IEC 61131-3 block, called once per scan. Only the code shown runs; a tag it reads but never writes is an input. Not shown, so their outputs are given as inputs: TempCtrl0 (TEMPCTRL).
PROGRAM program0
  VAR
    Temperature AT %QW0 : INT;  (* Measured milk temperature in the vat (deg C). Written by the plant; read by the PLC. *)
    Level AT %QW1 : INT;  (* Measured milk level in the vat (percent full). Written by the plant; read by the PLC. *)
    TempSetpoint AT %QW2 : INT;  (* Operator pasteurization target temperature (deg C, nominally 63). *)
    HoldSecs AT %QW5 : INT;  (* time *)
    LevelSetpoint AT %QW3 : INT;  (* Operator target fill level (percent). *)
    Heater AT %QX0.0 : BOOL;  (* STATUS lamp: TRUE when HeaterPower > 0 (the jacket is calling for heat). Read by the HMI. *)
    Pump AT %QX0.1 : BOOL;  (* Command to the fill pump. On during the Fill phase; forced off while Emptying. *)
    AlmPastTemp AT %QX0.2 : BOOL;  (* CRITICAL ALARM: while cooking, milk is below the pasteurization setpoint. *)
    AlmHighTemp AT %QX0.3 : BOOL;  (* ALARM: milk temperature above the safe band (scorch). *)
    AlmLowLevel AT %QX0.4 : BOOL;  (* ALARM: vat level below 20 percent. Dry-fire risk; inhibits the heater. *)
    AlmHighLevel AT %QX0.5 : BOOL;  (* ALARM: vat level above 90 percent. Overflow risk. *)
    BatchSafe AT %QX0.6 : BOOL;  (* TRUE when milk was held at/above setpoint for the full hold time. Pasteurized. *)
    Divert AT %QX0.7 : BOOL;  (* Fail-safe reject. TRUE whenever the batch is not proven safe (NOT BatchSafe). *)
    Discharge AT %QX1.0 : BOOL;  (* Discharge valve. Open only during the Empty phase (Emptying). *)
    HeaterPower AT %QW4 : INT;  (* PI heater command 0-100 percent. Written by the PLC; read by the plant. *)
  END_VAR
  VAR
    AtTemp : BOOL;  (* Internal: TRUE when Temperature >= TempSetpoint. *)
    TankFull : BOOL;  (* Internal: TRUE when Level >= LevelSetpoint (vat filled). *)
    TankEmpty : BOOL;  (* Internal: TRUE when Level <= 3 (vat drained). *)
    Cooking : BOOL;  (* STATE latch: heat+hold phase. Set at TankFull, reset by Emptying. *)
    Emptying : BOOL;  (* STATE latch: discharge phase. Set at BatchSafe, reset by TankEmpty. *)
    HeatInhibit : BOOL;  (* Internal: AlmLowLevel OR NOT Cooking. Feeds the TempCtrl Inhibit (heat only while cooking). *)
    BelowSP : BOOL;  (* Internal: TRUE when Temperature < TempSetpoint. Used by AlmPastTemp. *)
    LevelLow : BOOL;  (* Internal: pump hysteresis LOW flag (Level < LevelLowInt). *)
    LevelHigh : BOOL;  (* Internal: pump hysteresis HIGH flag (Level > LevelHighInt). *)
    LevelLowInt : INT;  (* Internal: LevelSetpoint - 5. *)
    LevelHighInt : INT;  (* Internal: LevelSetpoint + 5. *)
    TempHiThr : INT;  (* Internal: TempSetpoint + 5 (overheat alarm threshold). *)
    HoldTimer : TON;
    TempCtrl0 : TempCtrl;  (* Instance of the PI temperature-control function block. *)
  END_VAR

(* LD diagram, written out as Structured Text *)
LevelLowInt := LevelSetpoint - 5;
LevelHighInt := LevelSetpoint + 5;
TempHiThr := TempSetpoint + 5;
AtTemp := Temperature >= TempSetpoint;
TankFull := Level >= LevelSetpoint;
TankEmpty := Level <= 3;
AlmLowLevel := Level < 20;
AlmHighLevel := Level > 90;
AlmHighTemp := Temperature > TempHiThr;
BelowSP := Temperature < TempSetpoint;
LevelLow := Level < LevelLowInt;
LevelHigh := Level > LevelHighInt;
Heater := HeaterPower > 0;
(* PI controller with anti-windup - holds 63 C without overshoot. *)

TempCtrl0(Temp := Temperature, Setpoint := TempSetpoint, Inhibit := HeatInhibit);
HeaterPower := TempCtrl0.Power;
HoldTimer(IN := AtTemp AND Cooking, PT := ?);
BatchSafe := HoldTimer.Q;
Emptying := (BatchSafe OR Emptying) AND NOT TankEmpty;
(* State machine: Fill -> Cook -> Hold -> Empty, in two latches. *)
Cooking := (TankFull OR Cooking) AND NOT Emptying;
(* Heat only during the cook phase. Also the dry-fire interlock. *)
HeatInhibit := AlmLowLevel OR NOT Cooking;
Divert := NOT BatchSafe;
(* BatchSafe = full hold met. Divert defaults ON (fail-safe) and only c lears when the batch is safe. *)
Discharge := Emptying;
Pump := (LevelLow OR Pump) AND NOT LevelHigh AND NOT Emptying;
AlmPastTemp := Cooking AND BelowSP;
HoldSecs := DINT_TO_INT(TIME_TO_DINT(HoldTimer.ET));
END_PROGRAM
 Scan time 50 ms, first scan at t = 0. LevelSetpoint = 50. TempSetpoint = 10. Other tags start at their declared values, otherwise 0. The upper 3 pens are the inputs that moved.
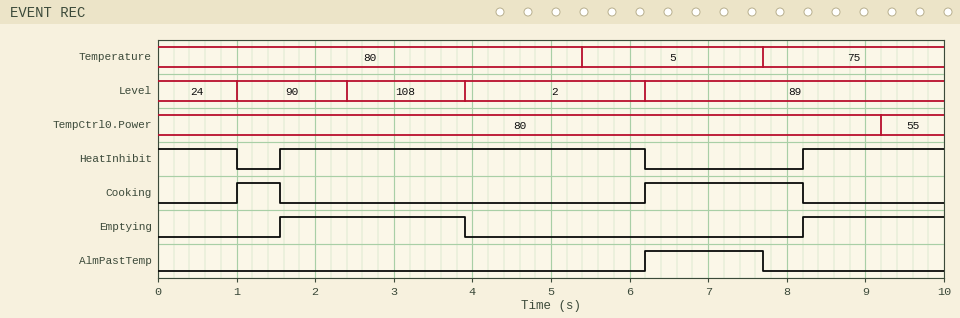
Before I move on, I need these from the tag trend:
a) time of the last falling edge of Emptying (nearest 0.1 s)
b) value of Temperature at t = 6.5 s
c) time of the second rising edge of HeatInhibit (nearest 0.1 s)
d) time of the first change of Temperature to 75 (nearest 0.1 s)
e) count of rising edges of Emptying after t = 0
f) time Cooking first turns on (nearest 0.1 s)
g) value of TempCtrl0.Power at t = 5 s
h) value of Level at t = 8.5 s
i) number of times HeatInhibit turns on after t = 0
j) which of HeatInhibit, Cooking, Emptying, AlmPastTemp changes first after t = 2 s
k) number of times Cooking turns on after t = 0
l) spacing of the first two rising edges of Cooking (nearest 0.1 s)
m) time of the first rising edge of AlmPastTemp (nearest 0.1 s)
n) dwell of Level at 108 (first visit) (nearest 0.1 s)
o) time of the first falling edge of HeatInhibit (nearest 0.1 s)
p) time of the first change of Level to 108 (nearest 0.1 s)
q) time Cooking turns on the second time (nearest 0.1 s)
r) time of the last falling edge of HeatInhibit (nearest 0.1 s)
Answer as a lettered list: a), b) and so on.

a) 3.9 s
b) 5
c) 8.2 s
d) 7.7 s
e) 2
f) 1.0 s
g) 80
h) 89
i) 2
j) Emptying
k) 2
l) 5.2 s
m) 6.2 s
n) 1.5 s
o) 1.0 s
p) 2.4 s
q) 6.2 s
r) 6.2 s
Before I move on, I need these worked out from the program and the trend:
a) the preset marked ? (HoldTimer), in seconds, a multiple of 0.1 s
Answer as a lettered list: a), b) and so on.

a) 0.5 s
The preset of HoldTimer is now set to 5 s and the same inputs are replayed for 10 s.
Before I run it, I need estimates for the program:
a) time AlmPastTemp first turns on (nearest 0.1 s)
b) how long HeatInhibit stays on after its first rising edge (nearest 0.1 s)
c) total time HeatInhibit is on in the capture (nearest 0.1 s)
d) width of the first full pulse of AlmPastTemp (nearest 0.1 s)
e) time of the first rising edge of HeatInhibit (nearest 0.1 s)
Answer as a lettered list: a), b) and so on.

a) 5.4 s
b) 2.3 s
c) 3.3 s
d) 2.3 s
e) 3.9 s
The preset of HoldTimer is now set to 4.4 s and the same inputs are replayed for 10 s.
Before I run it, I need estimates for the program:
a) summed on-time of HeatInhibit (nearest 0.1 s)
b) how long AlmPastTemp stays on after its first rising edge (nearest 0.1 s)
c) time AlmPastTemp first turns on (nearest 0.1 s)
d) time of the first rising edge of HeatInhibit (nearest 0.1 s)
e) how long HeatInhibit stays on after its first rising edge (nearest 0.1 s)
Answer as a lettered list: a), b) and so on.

a) 3.3 s
b) 2.3 s
c) 5.4 s
d) 3.9 s
e) 2.3 s
